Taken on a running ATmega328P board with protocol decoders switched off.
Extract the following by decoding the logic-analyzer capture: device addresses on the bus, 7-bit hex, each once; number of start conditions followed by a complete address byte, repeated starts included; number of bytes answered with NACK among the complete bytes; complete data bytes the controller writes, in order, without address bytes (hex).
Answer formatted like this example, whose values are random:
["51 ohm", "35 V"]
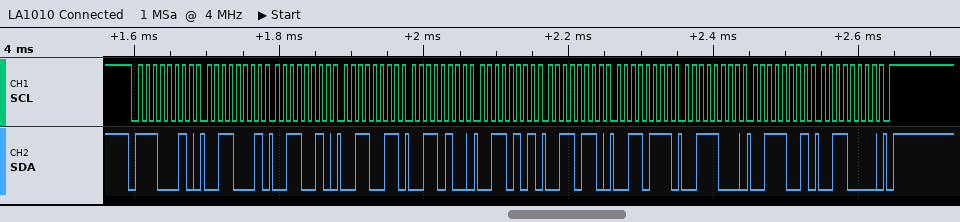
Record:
["0x71", "1", "0", "31 32 33 34 35 36 37 38 39 30"]
